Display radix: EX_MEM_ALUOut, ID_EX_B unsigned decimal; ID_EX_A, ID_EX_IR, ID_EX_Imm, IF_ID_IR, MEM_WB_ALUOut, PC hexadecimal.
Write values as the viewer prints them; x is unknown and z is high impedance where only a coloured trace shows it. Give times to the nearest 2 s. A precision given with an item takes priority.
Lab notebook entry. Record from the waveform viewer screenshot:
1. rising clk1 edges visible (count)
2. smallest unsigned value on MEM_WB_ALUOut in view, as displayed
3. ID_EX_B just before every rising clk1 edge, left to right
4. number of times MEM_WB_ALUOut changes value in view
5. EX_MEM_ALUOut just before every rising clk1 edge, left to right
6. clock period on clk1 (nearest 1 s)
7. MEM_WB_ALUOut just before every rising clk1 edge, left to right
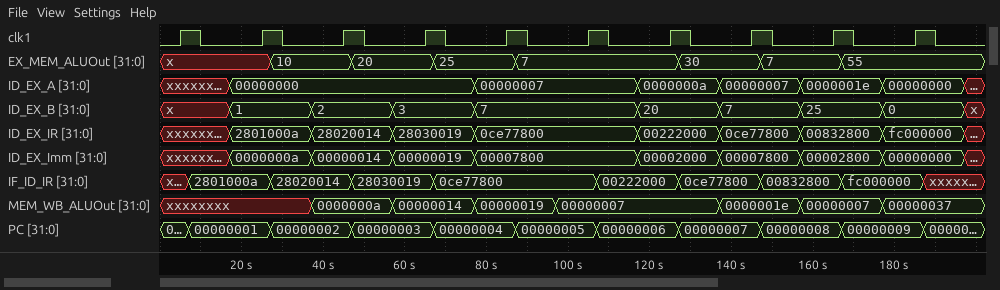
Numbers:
10
00000007
x, 1, 2, 3, 7, 7, 20, 7, 25, 0
7
x, x, 10, 20, 25, 7, 7, 30, 7, 55
20 s
xxxxxxxx, xxxxxxxx, 0000000a, 00000014, 00000019, 00000007, 00000007, 0000001e, 00000007, 00000037
